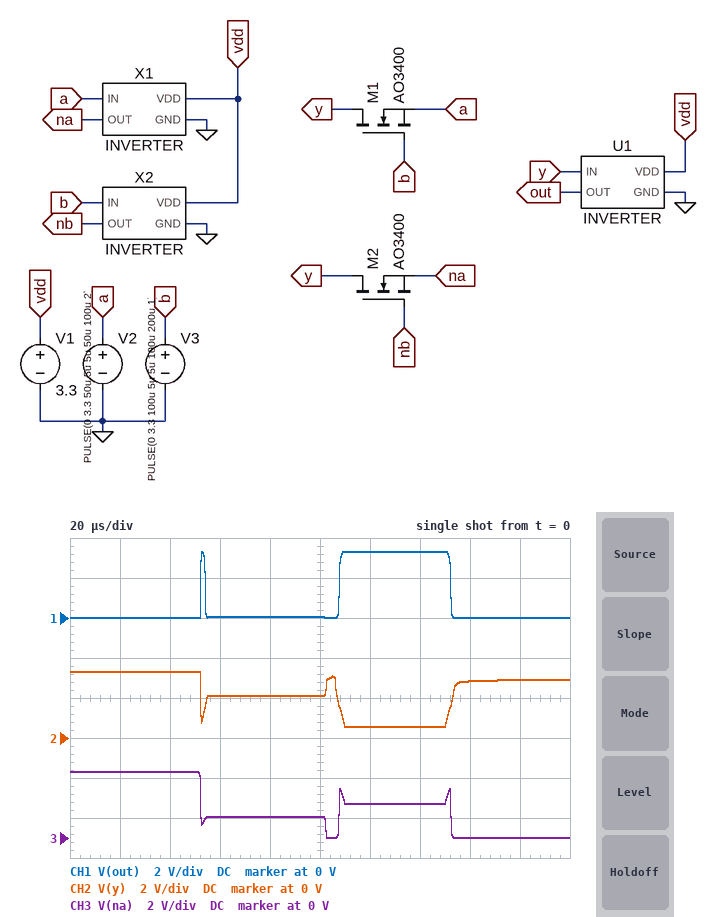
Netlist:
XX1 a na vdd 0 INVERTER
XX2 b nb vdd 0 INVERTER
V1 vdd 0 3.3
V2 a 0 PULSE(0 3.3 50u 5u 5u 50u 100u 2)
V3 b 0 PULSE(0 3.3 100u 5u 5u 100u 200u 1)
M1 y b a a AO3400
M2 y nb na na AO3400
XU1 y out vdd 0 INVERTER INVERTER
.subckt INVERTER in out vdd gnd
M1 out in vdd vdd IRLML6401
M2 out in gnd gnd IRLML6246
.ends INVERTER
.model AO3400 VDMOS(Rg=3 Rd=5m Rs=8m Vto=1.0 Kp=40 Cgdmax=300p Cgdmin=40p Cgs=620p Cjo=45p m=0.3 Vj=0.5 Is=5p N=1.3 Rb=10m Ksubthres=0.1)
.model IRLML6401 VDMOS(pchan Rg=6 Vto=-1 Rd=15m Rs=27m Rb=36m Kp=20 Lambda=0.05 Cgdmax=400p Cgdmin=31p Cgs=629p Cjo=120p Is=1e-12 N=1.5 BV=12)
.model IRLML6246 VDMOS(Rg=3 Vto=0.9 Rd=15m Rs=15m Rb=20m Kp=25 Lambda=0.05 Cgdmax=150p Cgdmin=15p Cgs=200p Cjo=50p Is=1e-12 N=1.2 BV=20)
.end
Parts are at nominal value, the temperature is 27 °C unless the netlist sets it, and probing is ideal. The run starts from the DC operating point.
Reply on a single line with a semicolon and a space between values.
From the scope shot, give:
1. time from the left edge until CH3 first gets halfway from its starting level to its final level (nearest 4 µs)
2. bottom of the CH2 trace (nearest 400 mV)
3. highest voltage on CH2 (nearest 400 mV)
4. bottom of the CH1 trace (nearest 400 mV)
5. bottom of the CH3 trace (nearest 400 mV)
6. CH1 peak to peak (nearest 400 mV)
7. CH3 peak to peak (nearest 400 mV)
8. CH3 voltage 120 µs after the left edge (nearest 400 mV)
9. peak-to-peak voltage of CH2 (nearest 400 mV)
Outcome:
52 µs; 400 mV; 3.2 V; 0 V; 0 V; 3.2 V; 3.2 V; 1.6 V; 2.8 V
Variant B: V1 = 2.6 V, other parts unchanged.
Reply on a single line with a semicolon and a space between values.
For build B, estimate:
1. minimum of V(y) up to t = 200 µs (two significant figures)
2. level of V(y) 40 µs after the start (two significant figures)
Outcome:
310 mV; 2.6 V
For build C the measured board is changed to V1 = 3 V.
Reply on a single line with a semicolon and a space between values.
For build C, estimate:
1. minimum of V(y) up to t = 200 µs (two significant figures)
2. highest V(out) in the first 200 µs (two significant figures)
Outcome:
430 mV; 3.0 V
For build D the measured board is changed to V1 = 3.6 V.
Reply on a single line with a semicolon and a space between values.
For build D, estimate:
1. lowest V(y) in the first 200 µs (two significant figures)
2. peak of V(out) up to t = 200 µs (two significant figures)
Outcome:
620 mV; 3.6 V
